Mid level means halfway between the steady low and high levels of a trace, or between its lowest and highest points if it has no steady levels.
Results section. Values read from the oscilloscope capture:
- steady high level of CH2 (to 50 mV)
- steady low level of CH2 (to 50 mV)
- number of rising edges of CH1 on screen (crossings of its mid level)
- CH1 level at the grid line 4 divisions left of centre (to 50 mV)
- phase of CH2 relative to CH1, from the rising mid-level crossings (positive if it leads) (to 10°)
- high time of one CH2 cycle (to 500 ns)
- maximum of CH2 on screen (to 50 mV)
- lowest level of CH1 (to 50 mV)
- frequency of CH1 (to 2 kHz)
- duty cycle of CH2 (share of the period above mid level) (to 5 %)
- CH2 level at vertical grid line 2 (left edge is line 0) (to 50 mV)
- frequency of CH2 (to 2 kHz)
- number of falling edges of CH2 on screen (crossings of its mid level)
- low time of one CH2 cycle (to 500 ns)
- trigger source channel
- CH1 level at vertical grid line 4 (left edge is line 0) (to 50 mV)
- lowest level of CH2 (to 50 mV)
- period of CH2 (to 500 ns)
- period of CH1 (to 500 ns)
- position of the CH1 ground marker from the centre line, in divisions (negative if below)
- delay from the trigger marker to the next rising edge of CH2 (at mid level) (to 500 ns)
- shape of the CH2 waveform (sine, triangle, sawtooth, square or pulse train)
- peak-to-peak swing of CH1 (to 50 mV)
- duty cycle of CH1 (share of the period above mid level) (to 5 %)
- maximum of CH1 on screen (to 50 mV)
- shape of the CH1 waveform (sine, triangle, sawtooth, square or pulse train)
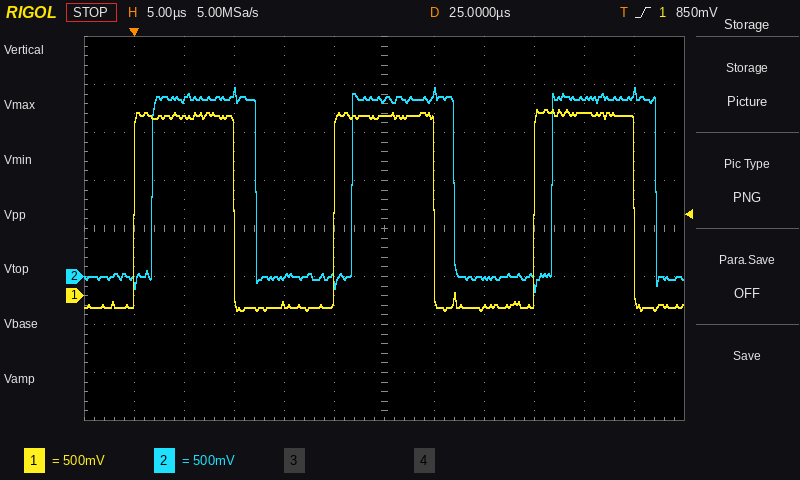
1.85 V
0 mV
3
1.85 V
-30°
10.5 µs
1.95 V
-150 mV
50 kHz
50 %
1.85 V
50 kHz
3
9.5 µs
CH1
-100 mV
-150 mV
20.0 µs
20.0 µs
-1.4 div
2.0 µs
square
2.10 V
50 %
1.95 V
square
